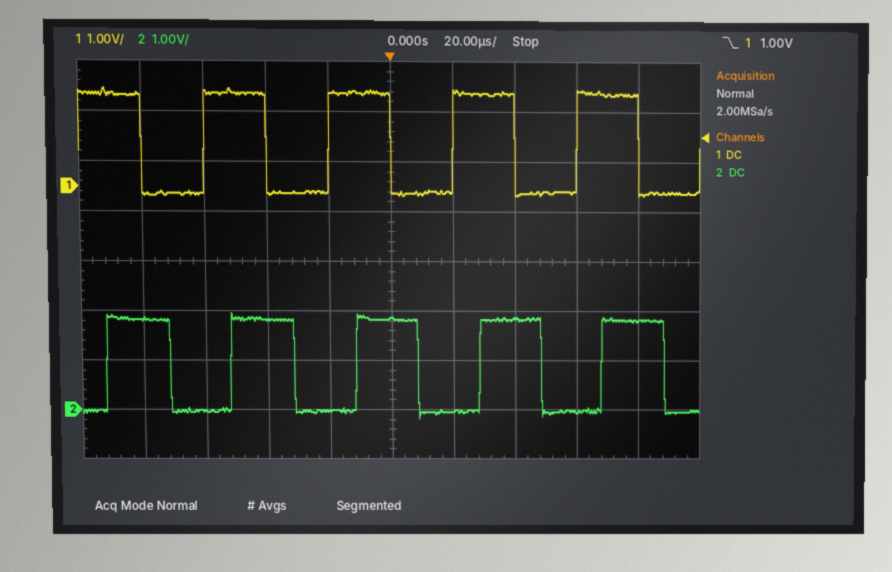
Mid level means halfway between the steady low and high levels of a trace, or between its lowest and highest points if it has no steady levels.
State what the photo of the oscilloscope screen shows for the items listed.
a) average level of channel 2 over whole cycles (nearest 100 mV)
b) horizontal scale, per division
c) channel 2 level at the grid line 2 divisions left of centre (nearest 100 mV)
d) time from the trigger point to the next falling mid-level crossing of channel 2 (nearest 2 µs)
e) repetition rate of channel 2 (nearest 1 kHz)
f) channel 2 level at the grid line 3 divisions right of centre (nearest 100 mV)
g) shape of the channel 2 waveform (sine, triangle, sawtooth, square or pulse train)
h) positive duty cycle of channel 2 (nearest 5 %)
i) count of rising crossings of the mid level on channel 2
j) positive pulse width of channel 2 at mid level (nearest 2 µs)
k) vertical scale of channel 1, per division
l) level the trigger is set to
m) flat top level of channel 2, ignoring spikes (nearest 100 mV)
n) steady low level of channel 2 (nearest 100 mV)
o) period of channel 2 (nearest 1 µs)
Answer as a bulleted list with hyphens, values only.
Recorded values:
- 900 mV
- 20 µs
- 1.8 V
- 8 µs
- 25 kHz
- 0.0 V
- square
- 50 %
- 5
- 20 µs
- 1 V
- 1.00 V
- 1.8 V
- 0.0 V
- 40 µs
